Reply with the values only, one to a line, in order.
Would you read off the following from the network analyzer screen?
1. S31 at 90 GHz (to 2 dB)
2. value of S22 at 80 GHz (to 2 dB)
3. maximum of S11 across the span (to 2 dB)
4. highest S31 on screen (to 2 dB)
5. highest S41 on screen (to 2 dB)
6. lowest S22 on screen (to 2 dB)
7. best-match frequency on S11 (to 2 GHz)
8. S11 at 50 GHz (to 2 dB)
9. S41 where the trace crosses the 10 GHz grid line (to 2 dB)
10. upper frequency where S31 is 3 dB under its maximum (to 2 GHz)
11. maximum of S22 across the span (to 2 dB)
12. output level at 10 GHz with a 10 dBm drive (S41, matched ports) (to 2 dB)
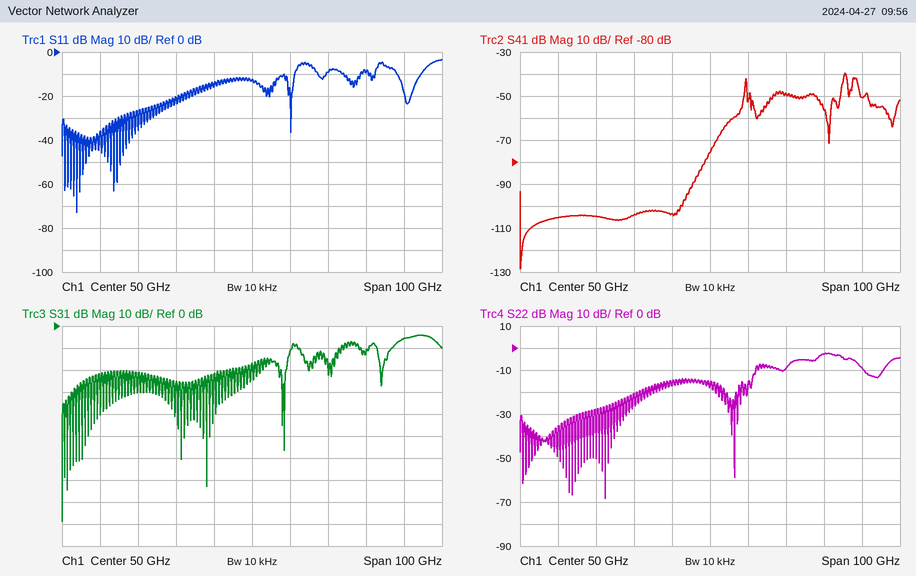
-6 dB
-2 dB
-4 dB
-4 dB
-40 dB
-68 dB
4 GHz
-12 dB
-106 dB
98 GHz
-2 dB
-96 dBm
